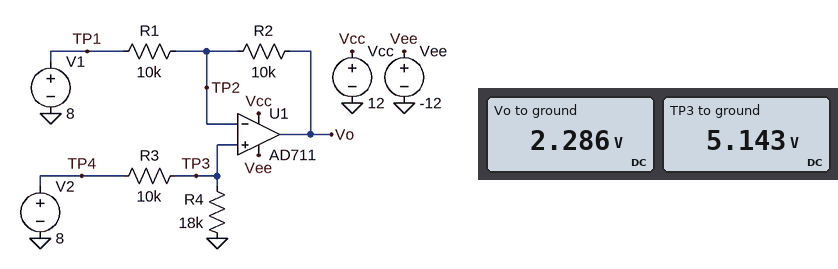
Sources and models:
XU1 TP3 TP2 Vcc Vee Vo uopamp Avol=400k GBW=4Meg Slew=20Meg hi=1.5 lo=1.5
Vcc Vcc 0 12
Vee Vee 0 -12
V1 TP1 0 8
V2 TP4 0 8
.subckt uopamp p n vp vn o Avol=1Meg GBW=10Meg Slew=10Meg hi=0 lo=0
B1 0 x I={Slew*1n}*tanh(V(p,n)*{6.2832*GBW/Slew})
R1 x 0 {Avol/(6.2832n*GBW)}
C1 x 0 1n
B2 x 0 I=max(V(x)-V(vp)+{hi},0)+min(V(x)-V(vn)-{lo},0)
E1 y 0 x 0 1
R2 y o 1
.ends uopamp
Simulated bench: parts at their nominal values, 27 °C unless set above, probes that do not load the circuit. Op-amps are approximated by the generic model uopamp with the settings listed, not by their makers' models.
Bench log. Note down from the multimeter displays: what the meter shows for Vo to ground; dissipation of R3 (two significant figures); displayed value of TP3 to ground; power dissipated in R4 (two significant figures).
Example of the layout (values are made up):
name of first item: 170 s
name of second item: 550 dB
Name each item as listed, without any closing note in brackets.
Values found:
what the meter shows for Vo to ground: 2.286 V
dissipation of R3: 820 µW
displayed value of TP3 to ground: 5.143 V
power dissipated in R4: 1.5 mW
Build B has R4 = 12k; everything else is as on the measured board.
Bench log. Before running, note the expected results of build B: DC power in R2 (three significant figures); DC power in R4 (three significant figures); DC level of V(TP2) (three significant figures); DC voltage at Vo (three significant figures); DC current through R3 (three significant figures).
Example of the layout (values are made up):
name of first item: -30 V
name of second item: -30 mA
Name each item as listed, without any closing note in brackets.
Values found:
DC power in R2: 1.32 mW
DC power in R4: 1.59 mW
DC level of V(TP2): 4.36 V
DC voltage at Vo: 727 mV
DC current through R3: 364 µA
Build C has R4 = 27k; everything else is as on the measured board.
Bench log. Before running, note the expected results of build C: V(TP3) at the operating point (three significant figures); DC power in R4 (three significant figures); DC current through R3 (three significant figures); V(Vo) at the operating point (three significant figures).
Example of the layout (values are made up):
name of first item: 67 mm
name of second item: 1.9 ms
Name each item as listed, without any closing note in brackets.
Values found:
V(TP3) at the operating point: 5.84 V
DC power in R4: 1.26 mW
DC current through R3: 216 µA
V(Vo) at the operating point: 3.68 V
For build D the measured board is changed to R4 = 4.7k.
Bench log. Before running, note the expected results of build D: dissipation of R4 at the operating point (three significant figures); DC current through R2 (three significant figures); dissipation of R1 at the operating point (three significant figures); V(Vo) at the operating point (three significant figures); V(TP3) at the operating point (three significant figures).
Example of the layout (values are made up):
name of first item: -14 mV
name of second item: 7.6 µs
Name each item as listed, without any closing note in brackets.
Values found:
dissipation of R4 at the operating point: 1.39 mW
DC current through R2: 544 µA
dissipation of R1 at the operating point: 2.96 mW
V(Vo) at the operating point: -2.88 V
V(TP3) at the operating point: 2.56 V
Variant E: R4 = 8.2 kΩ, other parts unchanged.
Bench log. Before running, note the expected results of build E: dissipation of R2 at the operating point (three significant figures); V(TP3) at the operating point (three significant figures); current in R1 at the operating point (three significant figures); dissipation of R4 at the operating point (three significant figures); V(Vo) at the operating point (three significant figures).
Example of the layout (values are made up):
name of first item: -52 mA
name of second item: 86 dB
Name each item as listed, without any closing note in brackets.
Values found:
dissipation of R2 at the operating point: 1.93 mW
V(TP3) at the operating point: 3.60 V
current in R1 at the operating point: 440 µA
dissipation of R4 at the operating point: 1.58 mW
V(Vo) at the operating point: -791 mV
